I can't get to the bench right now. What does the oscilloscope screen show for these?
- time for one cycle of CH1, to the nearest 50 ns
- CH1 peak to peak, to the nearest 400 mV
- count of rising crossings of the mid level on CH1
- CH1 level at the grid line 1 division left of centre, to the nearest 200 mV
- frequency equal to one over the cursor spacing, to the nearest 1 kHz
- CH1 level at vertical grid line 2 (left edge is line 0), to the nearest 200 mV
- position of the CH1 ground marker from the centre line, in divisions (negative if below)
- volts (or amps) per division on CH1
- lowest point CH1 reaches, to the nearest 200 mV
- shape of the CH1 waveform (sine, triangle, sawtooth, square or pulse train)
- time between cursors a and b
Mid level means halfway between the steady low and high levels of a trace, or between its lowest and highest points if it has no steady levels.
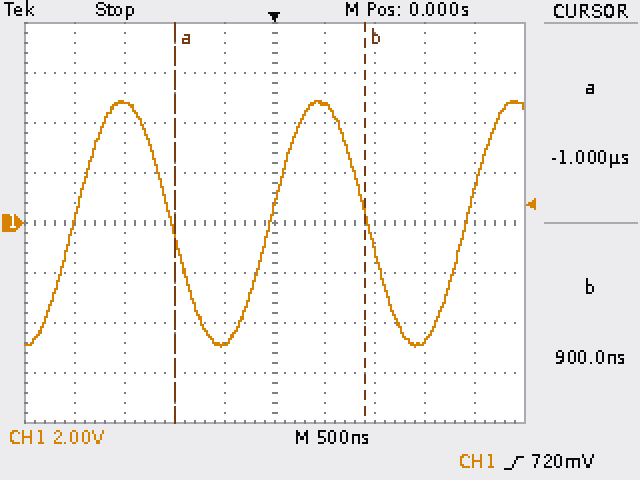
1.95 µs
10.0 V
3
-4.8 V
526 kHz
4.8 V
0.0 div
2 V
-5.0 V
sine
1.90 µs
